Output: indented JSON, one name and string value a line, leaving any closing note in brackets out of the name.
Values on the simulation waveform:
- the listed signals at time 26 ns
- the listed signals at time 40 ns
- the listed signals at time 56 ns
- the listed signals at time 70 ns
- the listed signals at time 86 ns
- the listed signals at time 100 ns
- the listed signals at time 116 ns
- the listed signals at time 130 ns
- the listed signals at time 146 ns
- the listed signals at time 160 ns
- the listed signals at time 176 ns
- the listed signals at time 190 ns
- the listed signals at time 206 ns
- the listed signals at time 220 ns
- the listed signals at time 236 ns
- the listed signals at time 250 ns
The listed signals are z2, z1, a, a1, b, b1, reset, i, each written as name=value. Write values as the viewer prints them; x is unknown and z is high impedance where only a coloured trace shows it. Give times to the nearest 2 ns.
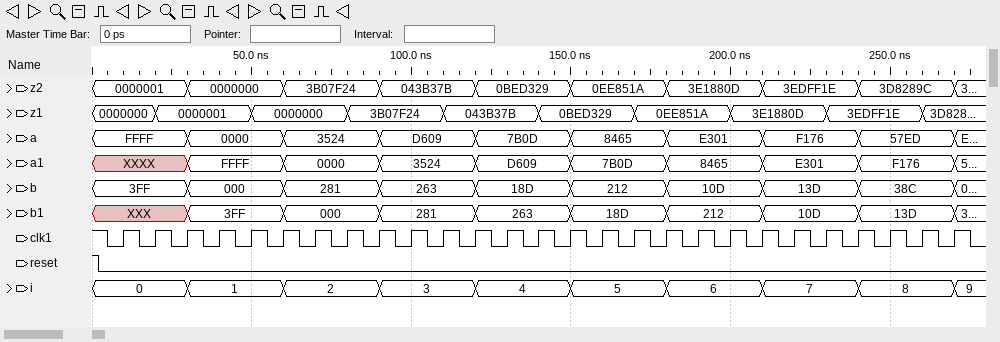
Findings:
{
  "the listed signals at time 26 ns": "z2=0000001, z1=0000001, a=FFFF, a1=XXXX, b=3FF, b1=XXX, reset=0, i=0",
  "the listed signals at time 40 ns": "z2=0000000, z1=0000001, a=0000, a1=FFFF, b=000, b1=3FF, reset=0, i=1",
  "the listed signals at time 56 ns": "z2=0000000, z1=0000000, a=0000, a1=FFFF, b=000, b1=3FF, reset=0, i=1",
  "the listed signals at time 70 ns": "z2=3B07F24, z1=0000000, a=3524, a1=0000, b=281, b1=000, reset=0, i=2",
  "the listed signals at time 86 ns": "z2=3B07F24, z1=3B07F24, a=3524, a1=0000, b=281, b1=000, reset=0, i=2",
  "the listed signals at time 100 ns": "z2=043B37B, z1=3B07F24, a=D609, a1=3524, b=263, b1=281, reset=0, i=3",
  "the listed signals at time 116 ns": "z2=043B37B, z1=043B37B, a=D609, a1=3524, b=263, b1=281, reset=0, i=3",
  "the listed signals at time 130 ns": "z2=0BED329, z1=043B37B, a=7B0D, a1=D609, b=18D, b1=263, reset=0, i=4",
  "the listed signals at time 146 ns": "z2=0BED329, z1=0BED329, a=7B0D, a1=D609, b=18D, b1=263, reset=0, i=4",
  "the listed signals at time 160 ns": "z2=0EE851A, z1=0BED329, a=8465, a1=7B0D, b=212, b1=18D, reset=0, i=5",
  "the listed signals at time 176 ns": "z2=0EE851A, z1=0EE851A, a=8465, a1=7B0D, b=212, b1=18D, reset=0, i=5",
  "the listed signals at time 190 ns": "z2=3E1880D, z1=0EE851A, a=E301, a1=8465, b=10D, b1=212, reset=0, i=6",
  "the listed signals at time 206 ns": "z2=3E1880D, z1=3E1880D, a=E301, a1=8465, b=10D, b1=212, reset=0, i=6",
  "the listed signals at time 220 ns": "z2=3EDFF1E, z1=3E1880D, a=F176, a1=E301, b=13D, b1=10D, reset=0, i=7",
  "the listed signals at time 236 ns": "z2=3EDFF1E, z1=3EDFF1E, a=F176, a1=E301, b=13D, b1=10D, reset=0, i=7",
  "the listed signals at time 250 ns": "z2=3D8289C, z1=3EDFF1E, a=57ED, a1=F176, b=38C, b1=13D, reset=0, i=8"
}
